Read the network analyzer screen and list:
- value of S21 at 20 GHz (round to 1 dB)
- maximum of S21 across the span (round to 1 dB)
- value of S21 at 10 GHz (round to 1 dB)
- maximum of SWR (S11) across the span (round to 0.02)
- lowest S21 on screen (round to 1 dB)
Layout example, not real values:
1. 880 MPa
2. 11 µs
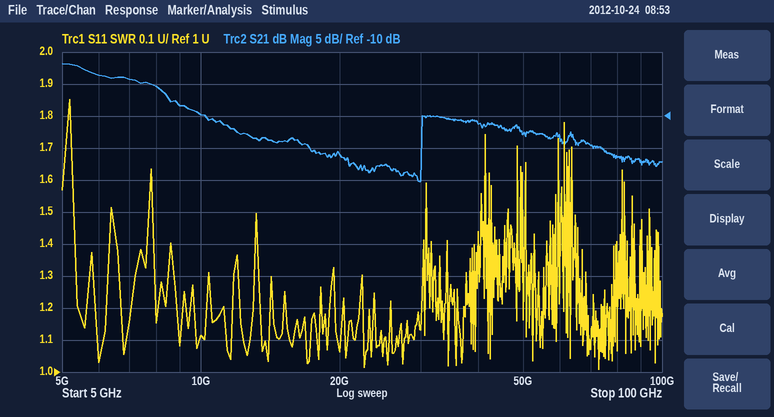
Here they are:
1. -16 dB
2. -2 dB
3. -10 dB
4. 1.86
5. -20 dB
